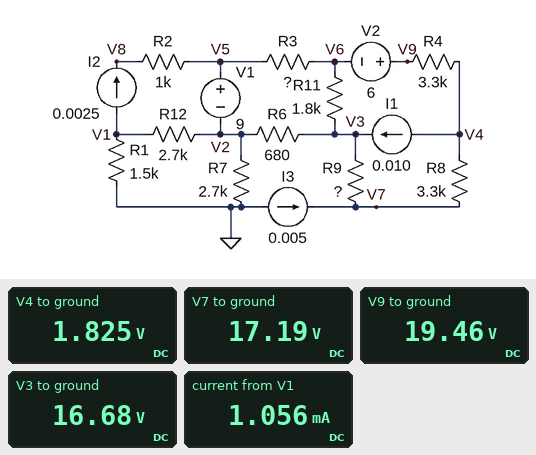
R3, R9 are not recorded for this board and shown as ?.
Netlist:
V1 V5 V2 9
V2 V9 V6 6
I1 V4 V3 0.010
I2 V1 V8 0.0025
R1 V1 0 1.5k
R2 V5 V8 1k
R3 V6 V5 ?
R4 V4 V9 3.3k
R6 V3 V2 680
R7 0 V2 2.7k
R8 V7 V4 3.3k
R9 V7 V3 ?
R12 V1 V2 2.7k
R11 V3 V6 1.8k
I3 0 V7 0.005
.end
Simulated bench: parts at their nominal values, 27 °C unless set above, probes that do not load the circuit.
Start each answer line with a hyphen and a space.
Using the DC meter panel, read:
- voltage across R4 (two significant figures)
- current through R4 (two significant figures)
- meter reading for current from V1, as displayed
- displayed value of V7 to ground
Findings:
- 18 V
- 5.3 mA
- 1.056 mA
- 17.19 V
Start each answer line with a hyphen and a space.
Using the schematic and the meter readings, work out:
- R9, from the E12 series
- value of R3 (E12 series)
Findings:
- 1.5 kΩ
- 1.8 kΩ
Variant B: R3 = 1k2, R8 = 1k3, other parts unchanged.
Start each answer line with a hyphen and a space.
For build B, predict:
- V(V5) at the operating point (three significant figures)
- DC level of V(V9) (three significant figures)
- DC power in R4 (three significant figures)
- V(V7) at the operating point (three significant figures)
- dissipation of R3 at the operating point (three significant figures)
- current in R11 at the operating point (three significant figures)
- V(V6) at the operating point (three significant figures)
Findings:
- 19.9 V
- 21.6 V
- 57.3 mW
- 15.4 V
- 15.2 mW
- 606 µA
- 15.6 V
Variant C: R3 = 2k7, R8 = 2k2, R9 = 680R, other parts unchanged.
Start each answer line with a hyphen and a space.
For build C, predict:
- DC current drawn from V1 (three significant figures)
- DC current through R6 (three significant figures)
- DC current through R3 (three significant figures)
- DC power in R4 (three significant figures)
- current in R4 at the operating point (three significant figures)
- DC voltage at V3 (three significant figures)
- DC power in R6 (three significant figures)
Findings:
- 157 µA
- 7.66 mA
- 2.66 mA
- 67.8 mW
- 4.53 mA
- 16.1 V
- 39.9 mW
